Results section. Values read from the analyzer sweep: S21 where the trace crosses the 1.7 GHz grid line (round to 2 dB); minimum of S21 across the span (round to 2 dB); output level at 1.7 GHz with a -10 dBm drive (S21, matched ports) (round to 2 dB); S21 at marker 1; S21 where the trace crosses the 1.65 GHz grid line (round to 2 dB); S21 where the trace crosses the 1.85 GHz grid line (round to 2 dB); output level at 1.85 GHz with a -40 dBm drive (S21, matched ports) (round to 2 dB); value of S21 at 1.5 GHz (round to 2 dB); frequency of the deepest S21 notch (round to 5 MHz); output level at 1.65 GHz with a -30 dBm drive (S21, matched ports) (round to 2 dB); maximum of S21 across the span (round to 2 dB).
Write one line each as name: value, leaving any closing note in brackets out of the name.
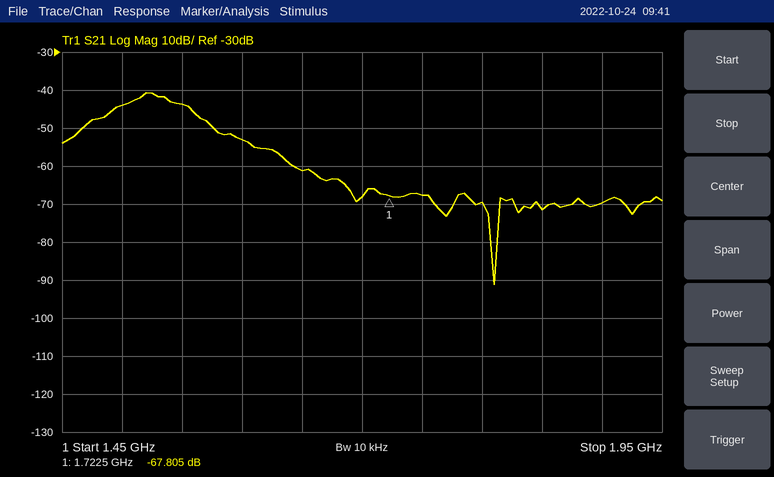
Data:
S21 where the trace crosses the 1.7 GHz grid line: -68 dB
minimum of S21 across the span: -92 dB
output level at 1.7 GHz with a -10 dBm drive (S21, matched ports): -78 dBm
S21 at marker 1: -67.805 dB
S21 where the trace crosses the 1.65 GHz grid line: -62 dB
S21 where the trace crosses the 1.85 GHz grid line: -72 dB
output level at 1.85 GHz with a -40 dBm drive (S21, matched ports): -112 dBm
value of S21 at 1.5 GHz: -44 dB
frequency of the deepest S21 notch: 1.810 GHz
output level at 1.65 GHz with a -30 dBm drive (S21, matched ports): -92 dBm
maximum of S21 across the span: -40 dB
